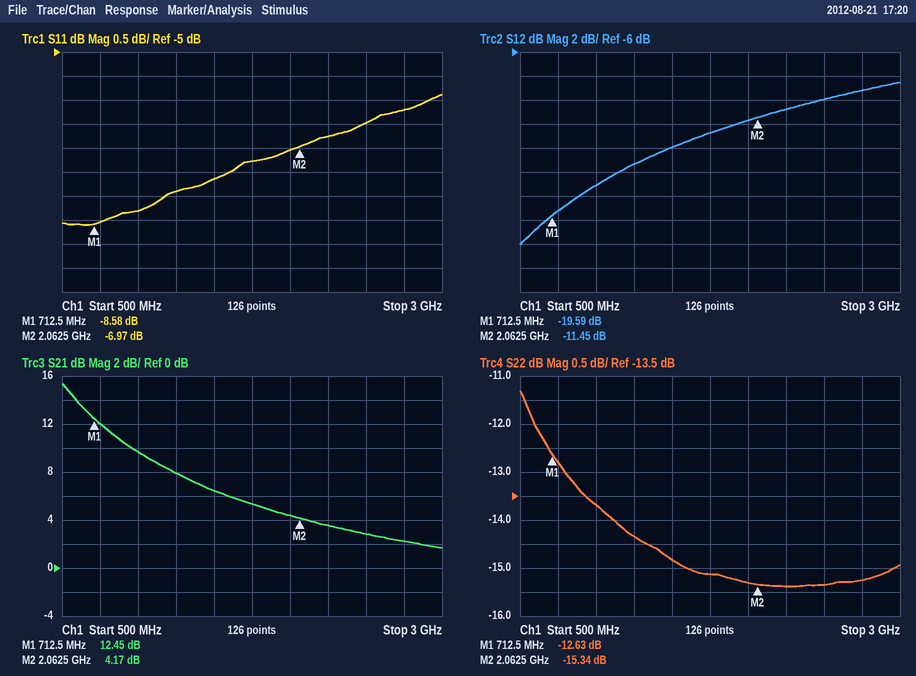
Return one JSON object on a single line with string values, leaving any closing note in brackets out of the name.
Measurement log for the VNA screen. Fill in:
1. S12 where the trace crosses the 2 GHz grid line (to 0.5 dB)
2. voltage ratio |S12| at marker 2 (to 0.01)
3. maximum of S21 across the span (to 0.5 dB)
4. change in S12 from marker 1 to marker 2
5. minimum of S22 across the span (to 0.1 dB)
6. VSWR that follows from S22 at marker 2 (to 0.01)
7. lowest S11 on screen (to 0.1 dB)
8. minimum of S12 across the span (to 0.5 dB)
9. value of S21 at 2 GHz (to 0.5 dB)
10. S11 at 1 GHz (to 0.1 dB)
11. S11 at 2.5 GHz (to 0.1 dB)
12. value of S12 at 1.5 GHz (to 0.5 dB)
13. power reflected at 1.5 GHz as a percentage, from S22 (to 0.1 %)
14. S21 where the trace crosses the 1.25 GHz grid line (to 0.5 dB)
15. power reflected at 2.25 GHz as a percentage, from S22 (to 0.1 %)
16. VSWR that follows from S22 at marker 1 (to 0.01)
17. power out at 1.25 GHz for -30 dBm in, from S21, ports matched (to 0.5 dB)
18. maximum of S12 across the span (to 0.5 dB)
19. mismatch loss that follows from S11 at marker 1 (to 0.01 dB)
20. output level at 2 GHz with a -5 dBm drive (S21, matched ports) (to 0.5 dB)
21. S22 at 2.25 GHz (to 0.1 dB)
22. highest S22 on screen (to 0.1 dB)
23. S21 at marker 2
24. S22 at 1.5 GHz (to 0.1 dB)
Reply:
{"S12 where the trace crosses the 2 GHz grid line": "-11.5 dB", "voltage ratio |S12| at marker 2": "0.27", "maximum of S21 across the span": "15.5 dB", "change in S12 from marker 1 to marker 2": "8.14 dB", "minimum of S22 across the span": "-15.4 dB", "VSWR that follows from S22 at marker 2": "1.41", "lowest S11 on screen": "-8.6 dB", "minimum of S12 across the span": "-22.0 dB", "value of S21 at 2 GHz": "4.5 dB", "S11 at 1 GHz": "-8.3 dB", "S11 at 2.5 GHz": "-6.5 dB", "value of S12 at 1.5 GHz": "-14.0 dB", "power reflected at 1.5 GHz as a percentage, from S22": "3.3 %", "S21 where the trace crosses the 1.25 GHz grid line": "8.0 dB", "power reflected at 2.25 GHz as a percentage, from S22": "2.9 %", "VSWR that follows from S22 at marker 1": "1.61", "power out at 1.25 GHz for -30 dBm in, from S21, ports matched": "-22.0 dBm", "maximum of S12 across the span": "-8.5 dB", "mismatch loss that follows from S11 at marker 1": "0.65 dB", "output level at 2 GHz with a -5 dBm drive (S21, matched ports)": "-0.5 dBm", "S22 at 2.25 GHz": "-15.4 dB", "highest S22 on screen": "-11.3 dB", "S21 at marker 2": "4.17 dB", "S22 at 1.5 GHz": "-14.8 dB"}
